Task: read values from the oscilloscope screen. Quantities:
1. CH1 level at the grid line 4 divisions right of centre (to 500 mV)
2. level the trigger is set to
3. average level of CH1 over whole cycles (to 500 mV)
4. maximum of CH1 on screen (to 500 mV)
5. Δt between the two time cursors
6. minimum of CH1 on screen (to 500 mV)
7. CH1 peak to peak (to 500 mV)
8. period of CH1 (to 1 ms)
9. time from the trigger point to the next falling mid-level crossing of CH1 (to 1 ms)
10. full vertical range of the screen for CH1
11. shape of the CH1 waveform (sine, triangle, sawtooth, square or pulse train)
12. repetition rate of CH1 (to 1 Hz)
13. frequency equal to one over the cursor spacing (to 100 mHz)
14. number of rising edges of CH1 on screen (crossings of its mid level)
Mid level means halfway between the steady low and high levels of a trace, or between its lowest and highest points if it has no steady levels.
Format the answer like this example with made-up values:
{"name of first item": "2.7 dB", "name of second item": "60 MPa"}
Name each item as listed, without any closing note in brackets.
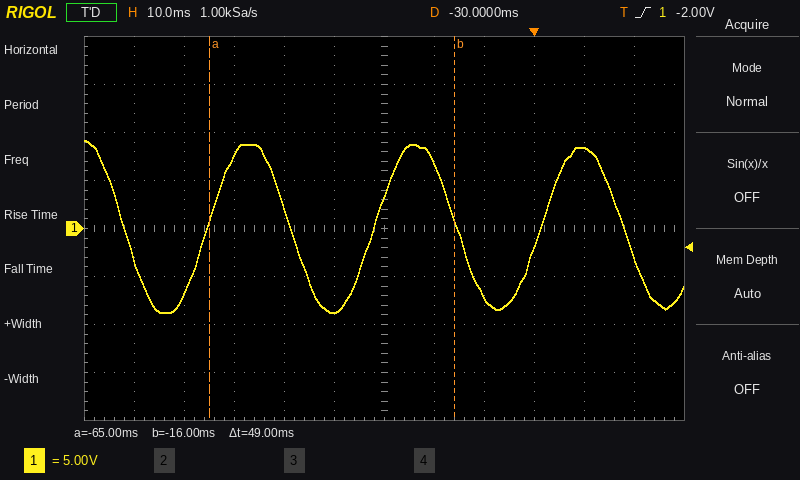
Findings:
{"CH1 level at the grid line 4 divisions right of centre": "8.5 V", "level the trigger is set to": "-2.00 V", "average level of CH1 over whole cycles": "0.0 V", "maximum of CH1 on screen": "9.0 V", "Δt between the two time cursors": "49 ms", "minimum of CH1 on screen": "-9.0 V", "CH1 peak to peak": "18.0 V", "period of CH1": "33 ms", "time from the trigger point to the next falling mid-level crossing of CH1": "18 ms", "full vertical range of the screen for CH1": "40 V", "shape of the CH1 waveform": "sine", "repetition rate of CH1": "30 Hz", "frequency equal to one over the cursor spacing": "20.4 Hz", "number of rising edges of CH1 on screen": "3"}
